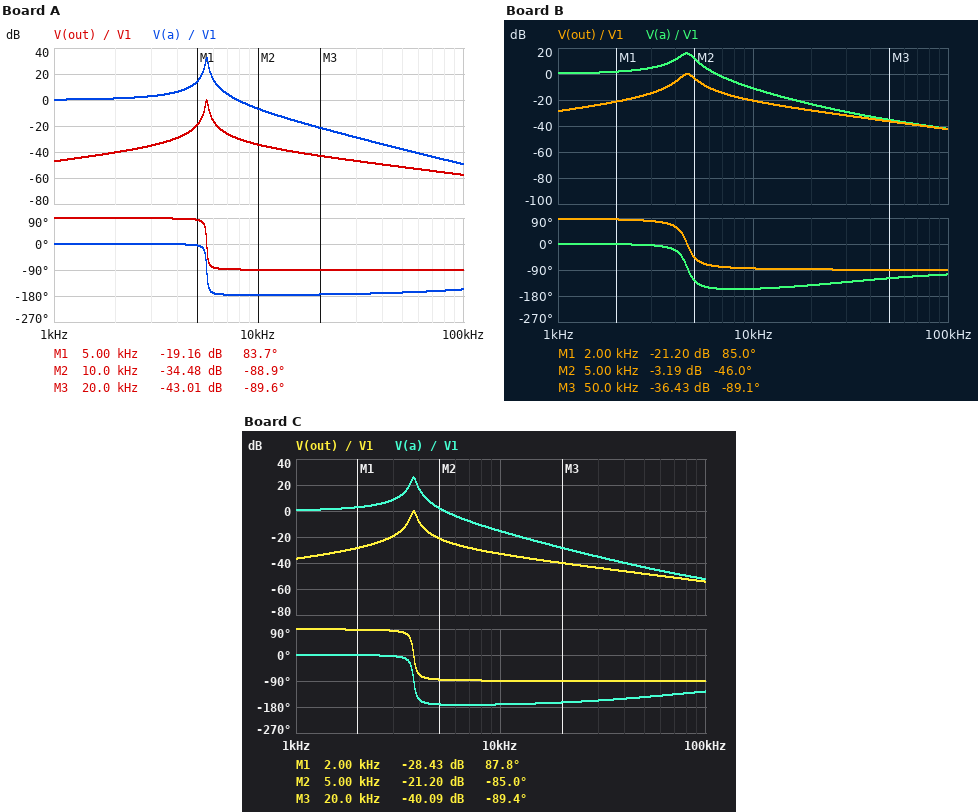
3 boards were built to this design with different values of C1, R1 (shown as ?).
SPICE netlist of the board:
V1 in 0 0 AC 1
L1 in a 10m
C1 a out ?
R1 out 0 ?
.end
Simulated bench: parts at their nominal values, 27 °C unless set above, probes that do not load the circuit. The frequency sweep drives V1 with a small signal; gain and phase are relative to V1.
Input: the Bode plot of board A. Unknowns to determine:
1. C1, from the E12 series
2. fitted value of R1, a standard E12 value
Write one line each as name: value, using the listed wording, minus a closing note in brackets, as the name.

C1, from the E12 series: 82 nF
fitted value of R1, a standard E12 value: 8.2 Ω
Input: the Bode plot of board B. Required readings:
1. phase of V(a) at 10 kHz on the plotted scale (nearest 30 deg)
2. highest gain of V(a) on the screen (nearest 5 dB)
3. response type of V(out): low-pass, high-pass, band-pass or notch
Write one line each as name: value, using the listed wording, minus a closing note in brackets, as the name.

phase of V(a) at 10 kHz on the plotted scale: -150 deg
highest gain of V(a) on the screen: 15 dB
response type of V(out): low-pass, high-pass, band-pass or notch: band-pass
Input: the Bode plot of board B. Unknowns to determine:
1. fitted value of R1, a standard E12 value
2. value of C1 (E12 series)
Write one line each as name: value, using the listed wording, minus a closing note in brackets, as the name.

fitted value of R1, a standard E12 value: 47 Ω
value of C1: 120 nF
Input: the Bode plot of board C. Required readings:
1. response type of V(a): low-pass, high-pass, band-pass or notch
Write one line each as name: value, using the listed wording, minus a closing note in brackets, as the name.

response type of V(a): low-pass, high-pass, band-pass or notch: low-pass
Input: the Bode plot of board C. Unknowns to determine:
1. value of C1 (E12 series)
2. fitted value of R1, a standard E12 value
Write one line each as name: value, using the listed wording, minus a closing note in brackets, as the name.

value of C1: 180 nF
fitted value of R1, a standard E12 value: 12 Ω
